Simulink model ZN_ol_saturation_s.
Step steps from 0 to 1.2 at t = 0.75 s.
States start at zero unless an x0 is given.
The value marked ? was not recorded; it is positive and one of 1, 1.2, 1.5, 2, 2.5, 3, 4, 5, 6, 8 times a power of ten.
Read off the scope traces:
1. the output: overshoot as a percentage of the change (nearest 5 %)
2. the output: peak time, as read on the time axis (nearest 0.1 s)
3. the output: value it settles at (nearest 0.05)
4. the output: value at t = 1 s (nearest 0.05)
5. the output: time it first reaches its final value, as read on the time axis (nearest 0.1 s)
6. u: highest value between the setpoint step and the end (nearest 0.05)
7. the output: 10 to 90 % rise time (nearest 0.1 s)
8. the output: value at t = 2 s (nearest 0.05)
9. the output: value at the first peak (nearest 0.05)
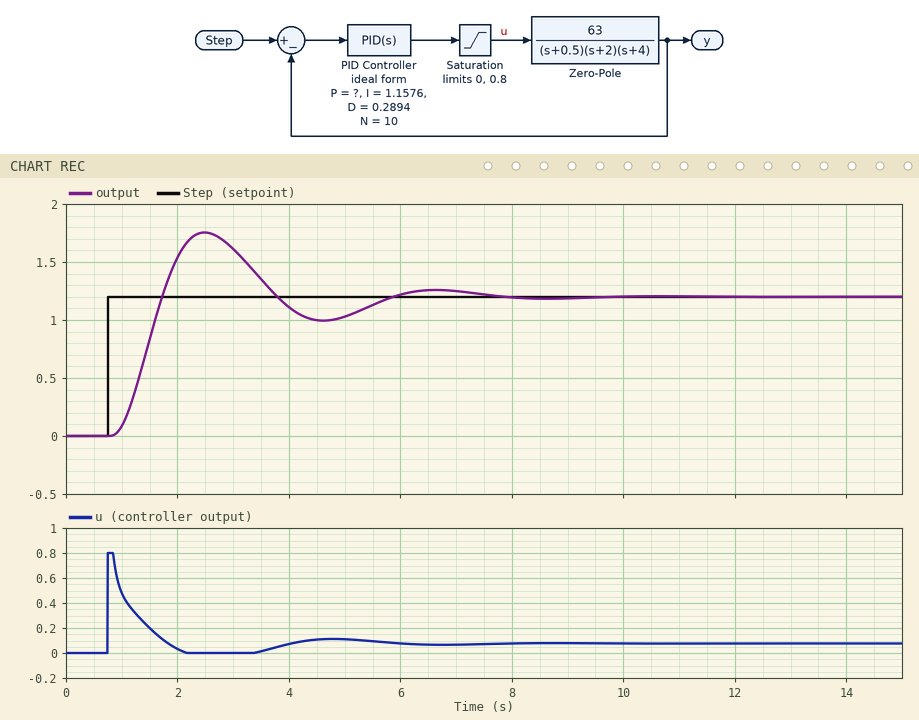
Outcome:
45 %
2.5 s
1.20
0.10
1.7 s
0.80
0.6 s
1.55
1.75
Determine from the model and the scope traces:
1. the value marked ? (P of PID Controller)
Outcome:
0.3
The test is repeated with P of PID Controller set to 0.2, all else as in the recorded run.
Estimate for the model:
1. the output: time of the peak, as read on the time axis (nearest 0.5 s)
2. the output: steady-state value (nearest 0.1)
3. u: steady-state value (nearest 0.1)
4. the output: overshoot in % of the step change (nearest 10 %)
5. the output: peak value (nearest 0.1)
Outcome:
3.0 s
1.2
0.1
40 %
1.7
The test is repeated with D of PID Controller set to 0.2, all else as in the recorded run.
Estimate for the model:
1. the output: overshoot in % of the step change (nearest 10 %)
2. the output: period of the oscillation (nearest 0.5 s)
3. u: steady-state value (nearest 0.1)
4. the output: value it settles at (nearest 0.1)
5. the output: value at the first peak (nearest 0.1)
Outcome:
60 %
4.5 s
0.1
1.2
1.9
